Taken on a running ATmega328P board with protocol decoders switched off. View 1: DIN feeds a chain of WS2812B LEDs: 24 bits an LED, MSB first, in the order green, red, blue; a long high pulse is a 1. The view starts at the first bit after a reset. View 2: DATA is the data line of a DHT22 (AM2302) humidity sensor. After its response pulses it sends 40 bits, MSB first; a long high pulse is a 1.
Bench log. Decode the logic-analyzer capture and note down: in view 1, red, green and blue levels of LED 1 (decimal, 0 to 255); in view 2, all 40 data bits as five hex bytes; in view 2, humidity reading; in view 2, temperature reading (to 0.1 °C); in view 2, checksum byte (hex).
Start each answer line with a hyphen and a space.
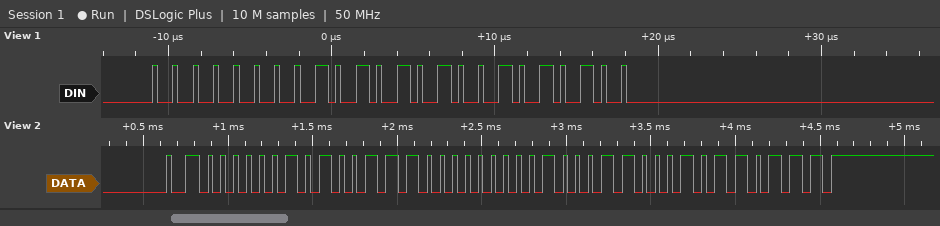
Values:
- 170, 0, 84
- 02 9C 01 18 B7
- 66.8 %
- 28.0 °C
- 0xB7
